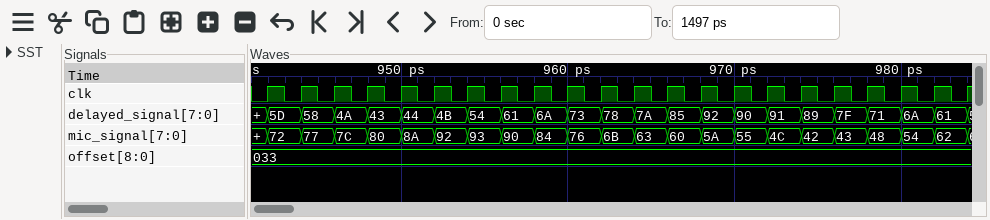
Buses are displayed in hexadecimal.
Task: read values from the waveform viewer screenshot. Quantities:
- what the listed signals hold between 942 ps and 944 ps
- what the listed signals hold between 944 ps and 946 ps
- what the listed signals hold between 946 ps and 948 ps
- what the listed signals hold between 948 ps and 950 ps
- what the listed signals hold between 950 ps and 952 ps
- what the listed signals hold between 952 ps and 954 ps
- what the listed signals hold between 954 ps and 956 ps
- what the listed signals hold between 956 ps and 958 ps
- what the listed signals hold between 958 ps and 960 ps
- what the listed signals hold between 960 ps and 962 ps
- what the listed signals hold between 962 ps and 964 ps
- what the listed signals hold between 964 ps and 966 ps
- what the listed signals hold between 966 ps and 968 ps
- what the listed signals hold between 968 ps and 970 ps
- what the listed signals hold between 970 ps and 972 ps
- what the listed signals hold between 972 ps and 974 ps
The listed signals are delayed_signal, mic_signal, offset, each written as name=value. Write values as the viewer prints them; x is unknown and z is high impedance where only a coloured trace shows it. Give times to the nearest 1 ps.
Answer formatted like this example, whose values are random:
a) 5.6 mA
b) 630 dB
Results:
a) delayed_signal=5D, mic_signal=72, offset=033
b) delayed_signal=58, mic_signal=77, offset=033
c) delayed_signal=4A, mic_signal=7C, offset=033
d) delayed_signal=43, mic_signal=80, offset=033
e) delayed_signal=44, mic_signal=8A, offset=033
f) delayed_signal=4B, mic_signal=92, offset=033
g) delayed_signal=54, mic_signal=93, offset=033
h) delayed_signal=61, mic_signal=90, offset=033
i) delayed_signal=6A, mic_signal=84, offset=033
j) delayed_signal=73, mic_signal=76, offset=033
k) delayed_signal=78, mic_signal=6B, offset=033
l) delayed_signal=7A, mic_signal=63, offset=033
m) delayed_signal=85, mic_signal=60, offset=033
n) delayed_signal=92, mic_signal=5A, offset=033
o) delayed_signal=90, mic_signal=55, offset=033
p) delayed_signal=91, mic_signal=4C, offset=033
